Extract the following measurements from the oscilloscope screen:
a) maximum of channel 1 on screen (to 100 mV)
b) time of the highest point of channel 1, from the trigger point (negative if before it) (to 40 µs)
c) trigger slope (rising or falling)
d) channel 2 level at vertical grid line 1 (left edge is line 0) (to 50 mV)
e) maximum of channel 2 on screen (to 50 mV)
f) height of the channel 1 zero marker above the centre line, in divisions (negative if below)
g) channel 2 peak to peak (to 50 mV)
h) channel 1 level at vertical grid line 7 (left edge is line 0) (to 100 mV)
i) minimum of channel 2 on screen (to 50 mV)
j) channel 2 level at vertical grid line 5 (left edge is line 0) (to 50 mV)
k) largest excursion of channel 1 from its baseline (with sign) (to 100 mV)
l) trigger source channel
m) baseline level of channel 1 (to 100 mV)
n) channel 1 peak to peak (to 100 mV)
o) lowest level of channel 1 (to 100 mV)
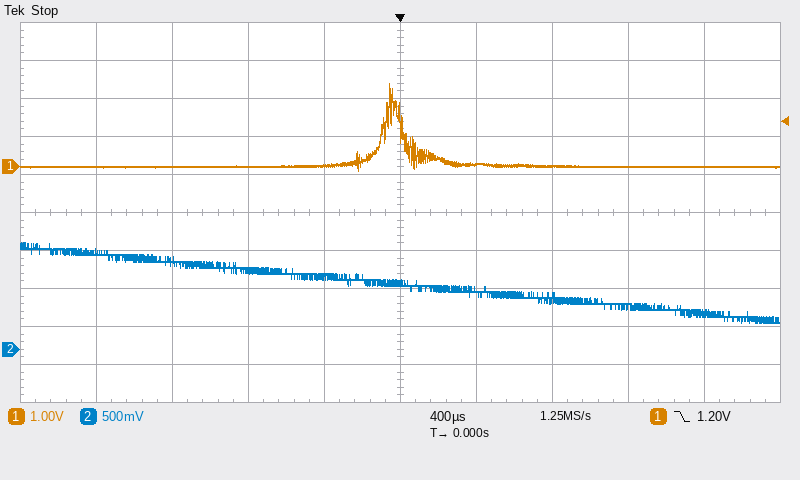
2.2 V
-40 µs
falling
1.30 V
1.40 V
+1.2 div
1.05 V
0.0 V
350 mV
900 mV
+2.2 V
channel 1
0.0 V
2.3 V
-100 mV
